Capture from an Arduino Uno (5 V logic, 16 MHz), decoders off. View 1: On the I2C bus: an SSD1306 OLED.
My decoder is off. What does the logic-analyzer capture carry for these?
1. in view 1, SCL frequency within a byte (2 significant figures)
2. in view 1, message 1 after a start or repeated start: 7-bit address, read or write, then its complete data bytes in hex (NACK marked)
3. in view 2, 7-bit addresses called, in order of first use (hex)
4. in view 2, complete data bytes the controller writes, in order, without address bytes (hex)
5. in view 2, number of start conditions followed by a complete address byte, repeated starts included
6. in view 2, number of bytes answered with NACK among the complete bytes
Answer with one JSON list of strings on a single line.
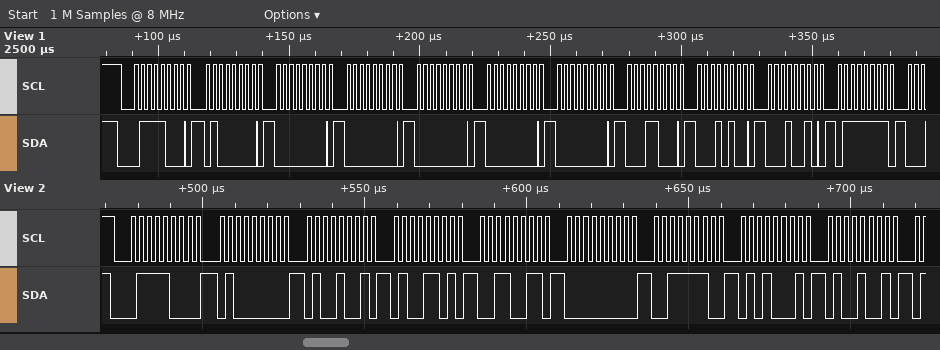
["400 kHz", "0x3C write: 40 00 00 00 00 00 18 14 12 7F", "0x3C", "40 49 4D 33 00 3E 51 49", "1", "0"]
